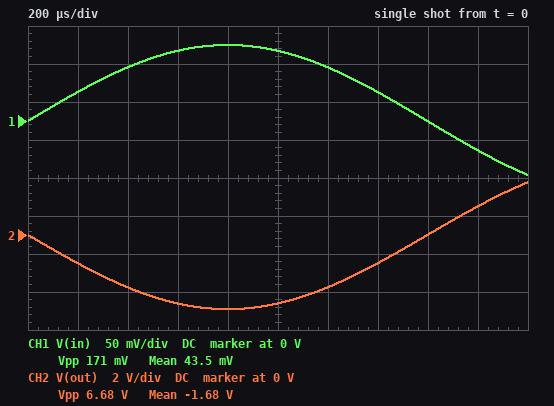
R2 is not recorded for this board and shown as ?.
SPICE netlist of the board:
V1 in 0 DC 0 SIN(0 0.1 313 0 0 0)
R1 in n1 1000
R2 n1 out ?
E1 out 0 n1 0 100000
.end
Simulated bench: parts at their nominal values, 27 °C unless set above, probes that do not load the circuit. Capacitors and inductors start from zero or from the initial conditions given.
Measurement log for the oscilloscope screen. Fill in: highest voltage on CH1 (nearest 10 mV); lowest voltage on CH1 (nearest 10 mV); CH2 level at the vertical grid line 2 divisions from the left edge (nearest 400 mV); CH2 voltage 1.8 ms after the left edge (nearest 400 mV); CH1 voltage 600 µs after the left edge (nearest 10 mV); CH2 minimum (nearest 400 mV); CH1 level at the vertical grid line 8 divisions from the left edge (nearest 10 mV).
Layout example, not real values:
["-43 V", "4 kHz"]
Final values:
["100 mV", "-70 mV", "-2.8 V", "1.6 V", "90 mV", "-4.0 V", "0 V"]
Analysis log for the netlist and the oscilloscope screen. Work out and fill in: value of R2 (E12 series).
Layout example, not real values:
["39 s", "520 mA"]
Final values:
["39 kΩ"]
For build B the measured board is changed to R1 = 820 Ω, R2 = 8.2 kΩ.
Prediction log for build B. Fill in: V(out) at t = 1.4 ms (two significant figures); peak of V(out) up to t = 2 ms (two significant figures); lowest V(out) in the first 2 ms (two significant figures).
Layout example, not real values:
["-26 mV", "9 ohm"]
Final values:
["-380 mV", "710 mV", "-1.0 V"]
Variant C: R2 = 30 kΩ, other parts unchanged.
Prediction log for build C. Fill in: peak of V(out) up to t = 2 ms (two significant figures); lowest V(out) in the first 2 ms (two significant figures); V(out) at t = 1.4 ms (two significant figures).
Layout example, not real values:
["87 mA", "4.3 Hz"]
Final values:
["2.1 V", "-3.0 V", "-1.1 V"]
